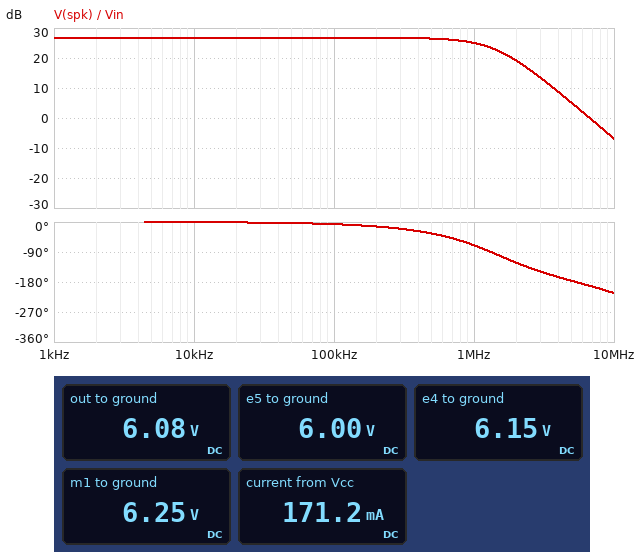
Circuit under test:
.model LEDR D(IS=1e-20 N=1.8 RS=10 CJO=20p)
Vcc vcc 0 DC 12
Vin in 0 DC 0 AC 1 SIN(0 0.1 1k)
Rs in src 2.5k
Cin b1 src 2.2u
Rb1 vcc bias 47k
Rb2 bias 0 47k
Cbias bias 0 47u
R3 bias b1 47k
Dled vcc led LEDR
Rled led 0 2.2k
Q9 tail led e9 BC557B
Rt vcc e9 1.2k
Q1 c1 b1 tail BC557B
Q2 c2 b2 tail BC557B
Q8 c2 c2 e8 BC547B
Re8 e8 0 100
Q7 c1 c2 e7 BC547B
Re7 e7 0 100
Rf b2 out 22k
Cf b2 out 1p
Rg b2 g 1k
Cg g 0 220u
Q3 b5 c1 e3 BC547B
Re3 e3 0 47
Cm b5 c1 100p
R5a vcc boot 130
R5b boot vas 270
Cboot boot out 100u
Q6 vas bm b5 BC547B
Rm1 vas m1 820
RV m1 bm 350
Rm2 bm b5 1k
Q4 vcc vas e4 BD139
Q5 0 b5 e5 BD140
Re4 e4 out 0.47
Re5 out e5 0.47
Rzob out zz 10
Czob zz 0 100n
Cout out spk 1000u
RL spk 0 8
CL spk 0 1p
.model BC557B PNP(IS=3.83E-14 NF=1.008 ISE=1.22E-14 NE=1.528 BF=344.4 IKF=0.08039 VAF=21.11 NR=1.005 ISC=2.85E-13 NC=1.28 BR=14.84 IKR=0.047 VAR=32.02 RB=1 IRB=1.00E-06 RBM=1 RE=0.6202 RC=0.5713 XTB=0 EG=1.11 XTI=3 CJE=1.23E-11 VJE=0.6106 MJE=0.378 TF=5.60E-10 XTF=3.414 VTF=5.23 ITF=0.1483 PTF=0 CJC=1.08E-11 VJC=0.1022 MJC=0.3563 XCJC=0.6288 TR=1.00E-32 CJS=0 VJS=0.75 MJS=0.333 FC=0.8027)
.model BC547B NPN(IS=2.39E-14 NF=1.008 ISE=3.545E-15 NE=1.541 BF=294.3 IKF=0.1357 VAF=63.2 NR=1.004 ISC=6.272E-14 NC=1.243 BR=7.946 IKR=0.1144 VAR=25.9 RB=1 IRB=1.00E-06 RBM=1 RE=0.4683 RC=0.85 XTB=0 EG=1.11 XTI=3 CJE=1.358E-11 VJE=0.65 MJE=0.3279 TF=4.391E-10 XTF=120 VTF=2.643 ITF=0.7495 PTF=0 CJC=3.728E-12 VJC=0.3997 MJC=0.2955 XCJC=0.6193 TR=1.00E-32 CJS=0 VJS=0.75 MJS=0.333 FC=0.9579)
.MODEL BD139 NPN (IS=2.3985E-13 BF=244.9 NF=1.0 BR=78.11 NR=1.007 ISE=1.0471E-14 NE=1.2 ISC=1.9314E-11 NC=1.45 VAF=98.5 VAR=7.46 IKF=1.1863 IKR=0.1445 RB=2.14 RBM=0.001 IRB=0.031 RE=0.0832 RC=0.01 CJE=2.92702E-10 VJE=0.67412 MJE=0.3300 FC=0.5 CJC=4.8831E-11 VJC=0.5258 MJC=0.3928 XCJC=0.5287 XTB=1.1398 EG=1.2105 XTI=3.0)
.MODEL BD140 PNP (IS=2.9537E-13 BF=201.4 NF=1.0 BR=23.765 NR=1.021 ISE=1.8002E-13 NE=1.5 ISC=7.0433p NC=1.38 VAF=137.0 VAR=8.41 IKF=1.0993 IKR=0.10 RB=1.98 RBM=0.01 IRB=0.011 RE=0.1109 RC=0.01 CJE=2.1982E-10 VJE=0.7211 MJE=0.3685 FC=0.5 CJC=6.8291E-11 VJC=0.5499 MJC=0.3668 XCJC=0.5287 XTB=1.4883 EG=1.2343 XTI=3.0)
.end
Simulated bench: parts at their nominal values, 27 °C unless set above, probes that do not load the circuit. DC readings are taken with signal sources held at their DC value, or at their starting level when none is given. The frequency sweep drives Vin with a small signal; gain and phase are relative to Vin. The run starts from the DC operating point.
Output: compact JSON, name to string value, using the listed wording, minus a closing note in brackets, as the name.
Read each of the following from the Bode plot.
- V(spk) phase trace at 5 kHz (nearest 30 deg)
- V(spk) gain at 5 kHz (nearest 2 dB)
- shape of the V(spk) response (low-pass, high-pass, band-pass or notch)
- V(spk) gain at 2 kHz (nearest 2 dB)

{"V(spk) phase trace at 5 kHz": "0 deg", "V(spk) gain at 5 kHz": "26 dB", "shape of the V(spk) response": "low-pass", "V(spk) gain at 2 kHz": "26 dB"}
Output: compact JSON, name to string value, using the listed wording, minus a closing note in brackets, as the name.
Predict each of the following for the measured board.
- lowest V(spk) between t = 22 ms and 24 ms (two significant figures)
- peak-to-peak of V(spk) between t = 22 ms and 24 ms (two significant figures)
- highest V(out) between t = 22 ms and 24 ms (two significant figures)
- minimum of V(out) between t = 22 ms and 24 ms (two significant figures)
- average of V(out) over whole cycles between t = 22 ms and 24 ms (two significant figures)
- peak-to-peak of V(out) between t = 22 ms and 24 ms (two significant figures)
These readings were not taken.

{"lowest V(spk) between t = 22 ms and 24 ms": "-2.2 V", "peak-to-peak of V(spk) between t = 22 ms and 24 ms": "4.3 V", "highest V(out) between t = 22 ms and 24 ms": "8.2 V", "minimum of V(out) between t = 22 ms and 24 ms": "3.9 V", "average of V(out) over whole cycles between t = 22 ms and 24 ms": "6.1 V", "peak-to-peak of V(out) between t = 22 ms and 24 ms": "4.3 V"}
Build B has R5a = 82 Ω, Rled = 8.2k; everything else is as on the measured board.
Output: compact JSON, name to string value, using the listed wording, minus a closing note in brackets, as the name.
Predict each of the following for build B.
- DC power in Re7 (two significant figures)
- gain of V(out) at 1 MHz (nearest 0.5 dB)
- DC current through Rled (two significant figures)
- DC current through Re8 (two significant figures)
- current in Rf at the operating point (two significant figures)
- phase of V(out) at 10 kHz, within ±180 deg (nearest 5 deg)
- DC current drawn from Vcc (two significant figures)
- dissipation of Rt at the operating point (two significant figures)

{"DC power in Re7": "23 µW", "gain of V(out) at 1 MHz": "24.5 dB", "DC current through Rled": "1.2 mA", "DC current through Re8": "480 µA", "current in Rf at the operating point": "1.2 µA", "phase of V(out) at 10 kHz, within ±180 deg": "0 deg", "DC current drawn from Vcc": "180 mA", "dissipation of Rt at the operating point": "1.2 mW"}
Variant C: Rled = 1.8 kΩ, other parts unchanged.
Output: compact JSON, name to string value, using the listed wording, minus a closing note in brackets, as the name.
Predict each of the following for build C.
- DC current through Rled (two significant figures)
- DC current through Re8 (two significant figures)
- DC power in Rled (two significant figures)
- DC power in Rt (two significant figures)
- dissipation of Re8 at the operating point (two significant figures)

{"DC current through Rled": "5.6 mA", "DC current through Re8": "530 µA", "DC power in Rled": "56 mW", "DC power in Rt": "1.5 mW", "dissipation of Re8 at the operating point": "28 µW"}
